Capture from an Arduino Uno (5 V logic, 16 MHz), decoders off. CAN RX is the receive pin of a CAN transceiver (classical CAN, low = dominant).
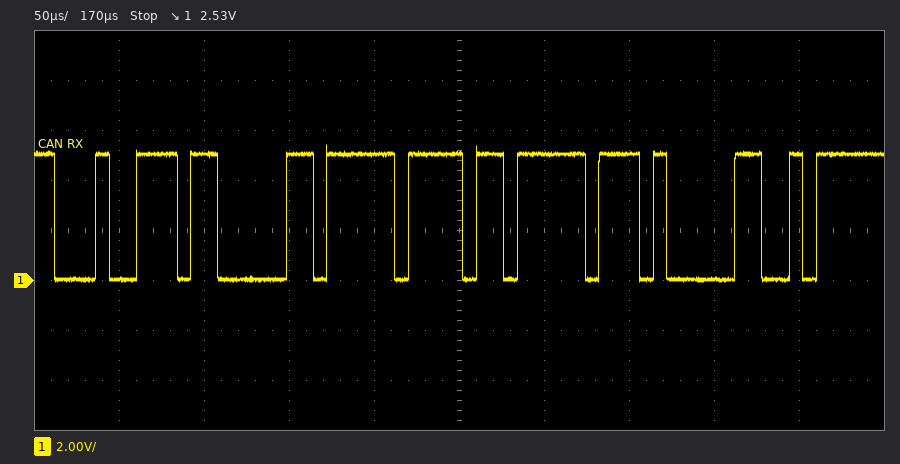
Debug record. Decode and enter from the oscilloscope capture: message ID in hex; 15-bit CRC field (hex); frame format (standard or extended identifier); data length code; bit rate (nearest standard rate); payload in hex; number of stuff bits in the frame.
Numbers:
0x13B
0x7D04
standard
2
125 kbit/s
FF B7
4
